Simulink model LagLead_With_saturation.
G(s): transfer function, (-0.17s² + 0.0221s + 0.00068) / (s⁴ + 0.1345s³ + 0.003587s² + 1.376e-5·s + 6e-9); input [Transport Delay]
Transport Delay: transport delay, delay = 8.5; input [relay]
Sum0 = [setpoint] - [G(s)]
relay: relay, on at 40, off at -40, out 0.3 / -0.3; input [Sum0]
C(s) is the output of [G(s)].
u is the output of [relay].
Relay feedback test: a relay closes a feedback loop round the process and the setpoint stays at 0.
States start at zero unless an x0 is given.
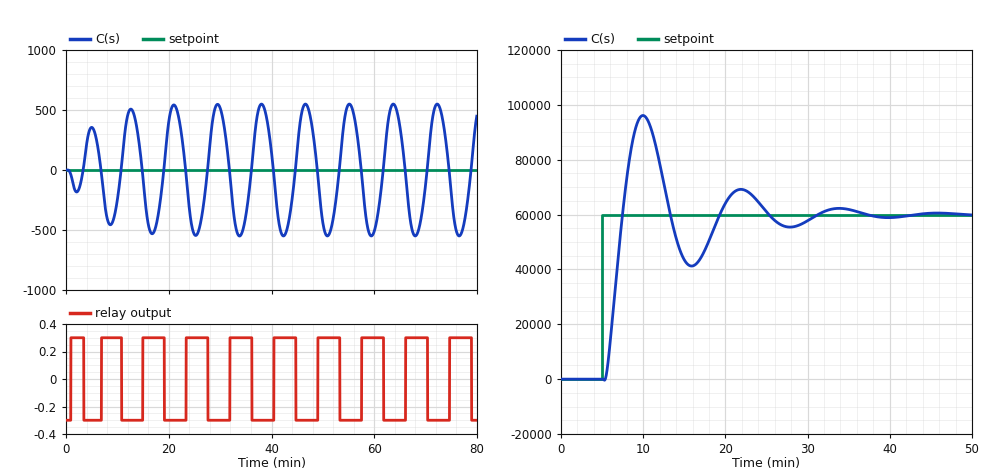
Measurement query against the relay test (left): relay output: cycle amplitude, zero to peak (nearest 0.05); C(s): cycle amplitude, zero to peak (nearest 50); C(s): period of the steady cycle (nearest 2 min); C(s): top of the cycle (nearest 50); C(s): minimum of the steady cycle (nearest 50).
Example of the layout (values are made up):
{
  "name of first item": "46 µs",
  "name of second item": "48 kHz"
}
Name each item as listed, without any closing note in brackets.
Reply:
{
  "relay output: cycle amplitude, zero to peak": "0.30",
  "C(s): cycle amplitude, zero to peak": "550",
  "C(s): period of the steady cycle": "8 min",
  "C(s): top of the cycle": "550",
  "C(s): minimum of the steady cycle": "-550"
}
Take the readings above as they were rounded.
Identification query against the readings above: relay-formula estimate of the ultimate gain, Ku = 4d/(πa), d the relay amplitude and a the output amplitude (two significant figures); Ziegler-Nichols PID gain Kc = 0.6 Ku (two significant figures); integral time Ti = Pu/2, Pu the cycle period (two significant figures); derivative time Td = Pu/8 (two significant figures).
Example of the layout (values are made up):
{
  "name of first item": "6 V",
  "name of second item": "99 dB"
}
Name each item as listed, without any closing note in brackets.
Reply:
{
  "relay-formula estimate of the ultimate gain, Ku = 4d/(πa), d the relay amplitude and a the output amplitude": "0.00069",
  "Ziegler-Nichols PID gain Kc = 0.6 Ku": "0.00041",
  "integral time Ti = Pu/2, Pu the cycle period": "4.0 min",
  "derivative time Td = Pu/8": "1.0 min"
}
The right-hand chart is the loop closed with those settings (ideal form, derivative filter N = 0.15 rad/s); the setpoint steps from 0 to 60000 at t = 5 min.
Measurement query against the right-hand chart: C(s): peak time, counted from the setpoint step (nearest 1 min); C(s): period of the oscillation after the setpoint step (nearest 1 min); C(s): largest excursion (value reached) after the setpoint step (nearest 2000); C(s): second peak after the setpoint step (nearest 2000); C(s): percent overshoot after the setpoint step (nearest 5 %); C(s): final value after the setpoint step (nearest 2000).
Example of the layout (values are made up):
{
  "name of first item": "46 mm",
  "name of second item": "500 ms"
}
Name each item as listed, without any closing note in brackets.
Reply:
{
  "C(s): peak time, counted from the setpoint step": "5 min",
  "C(s): period of the oscillation after the setpoint step": "12 min",
  "C(s): largest excursion (value reached) after the setpoint step": "96000",
  "C(s): second peak after the setpoint step": "70000",
  "C(s): percent overshoot after the setpoint step": "60 %",
  "C(s): final value after the setpoint step": "60000"
}
